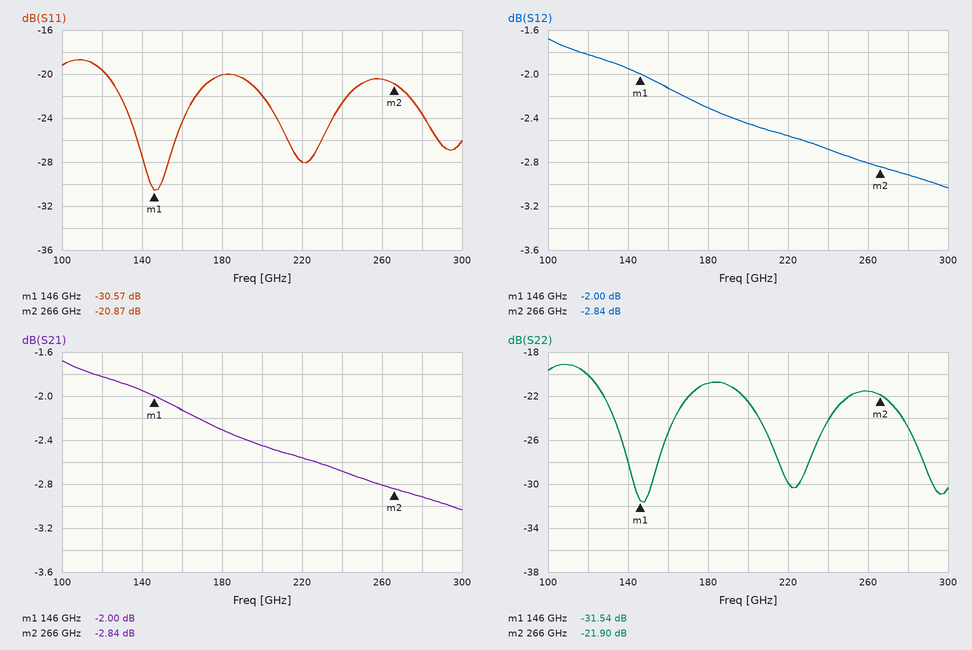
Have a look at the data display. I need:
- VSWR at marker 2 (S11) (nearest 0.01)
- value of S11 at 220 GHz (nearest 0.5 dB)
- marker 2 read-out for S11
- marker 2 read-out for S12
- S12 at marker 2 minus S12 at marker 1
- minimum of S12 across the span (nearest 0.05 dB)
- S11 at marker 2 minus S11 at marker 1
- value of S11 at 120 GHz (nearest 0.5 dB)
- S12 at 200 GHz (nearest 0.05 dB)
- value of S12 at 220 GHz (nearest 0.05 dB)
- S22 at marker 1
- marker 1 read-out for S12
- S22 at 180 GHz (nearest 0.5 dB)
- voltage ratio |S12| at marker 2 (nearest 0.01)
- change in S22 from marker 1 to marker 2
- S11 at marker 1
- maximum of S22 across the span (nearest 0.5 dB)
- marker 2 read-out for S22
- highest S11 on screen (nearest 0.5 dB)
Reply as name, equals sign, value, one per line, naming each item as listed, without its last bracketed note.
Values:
VSWR at marker 2 (S11) = 1.20
value of S11 at 220 GHz = -28.0 dB
marker 2 read-out for S11 = -20.87 dB
marker 2 read-out for S12 = -2.84 dB
S12 at marker 2 minus S12 at marker 1 = -0.84 dB
minimum of S12 across the span = -3.05 dB
S11 at marker 2 minus S11 at marker 1 = 9.70 dB
value of S11 at 120 GHz = -19.5 dB
S12 at 200 GHz = -2.45 dB
value of S12 at 220 GHz = -2.55 dB
S22 at marker 1 = -31.54 dB
marker 1 read-out for S12 = -2.00 dB
S22 at 180 GHz = -21.0 dB
voltage ratio |S12| at marker 2 = 0.72
change in S22 from marker 1 to marker 2 = 9.64 dB
S11 at marker 1 = -30.57 dB
maximum of S22 across the span = -19.0 dB
marker 2 read-out for S22 = -21.90 dB
highest S11 on screen = -18.5 dB
